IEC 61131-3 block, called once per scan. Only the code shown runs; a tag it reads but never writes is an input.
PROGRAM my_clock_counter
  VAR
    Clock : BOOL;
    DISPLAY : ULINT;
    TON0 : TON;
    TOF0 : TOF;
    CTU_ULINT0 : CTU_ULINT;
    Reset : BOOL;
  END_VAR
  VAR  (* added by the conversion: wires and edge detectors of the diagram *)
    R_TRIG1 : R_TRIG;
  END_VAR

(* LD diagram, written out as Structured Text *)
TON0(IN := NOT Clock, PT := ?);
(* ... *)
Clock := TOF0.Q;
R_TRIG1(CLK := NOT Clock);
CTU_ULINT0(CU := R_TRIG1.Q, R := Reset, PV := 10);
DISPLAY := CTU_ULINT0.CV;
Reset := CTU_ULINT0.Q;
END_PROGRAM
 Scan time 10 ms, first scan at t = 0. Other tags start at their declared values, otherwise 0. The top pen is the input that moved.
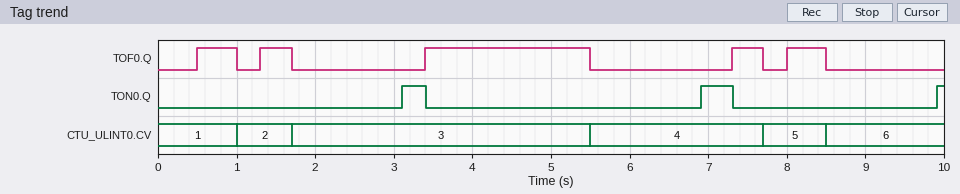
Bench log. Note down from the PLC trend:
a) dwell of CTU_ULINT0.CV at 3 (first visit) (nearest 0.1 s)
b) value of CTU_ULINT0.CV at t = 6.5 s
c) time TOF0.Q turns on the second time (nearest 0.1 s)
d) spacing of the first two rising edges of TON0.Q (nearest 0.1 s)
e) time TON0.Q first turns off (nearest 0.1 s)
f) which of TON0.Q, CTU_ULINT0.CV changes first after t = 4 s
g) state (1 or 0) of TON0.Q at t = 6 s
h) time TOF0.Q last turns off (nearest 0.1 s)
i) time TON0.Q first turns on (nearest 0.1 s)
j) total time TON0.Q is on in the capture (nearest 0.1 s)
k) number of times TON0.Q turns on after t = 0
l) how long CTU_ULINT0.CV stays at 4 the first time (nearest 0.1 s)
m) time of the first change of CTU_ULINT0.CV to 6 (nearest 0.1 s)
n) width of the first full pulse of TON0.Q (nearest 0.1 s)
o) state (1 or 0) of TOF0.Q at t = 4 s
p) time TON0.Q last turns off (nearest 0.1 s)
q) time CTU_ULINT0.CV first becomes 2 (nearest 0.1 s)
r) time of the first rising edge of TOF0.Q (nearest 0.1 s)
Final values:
3.8 s
4
1.3 s
3.8 s
3.4 s
CTU_ULINT0.CV
0
8.5 s
3.1 s
0.8 s
3
2.2 s
8.5 s
0.3 s
1
7.3 s
1.0 s
0.5 s
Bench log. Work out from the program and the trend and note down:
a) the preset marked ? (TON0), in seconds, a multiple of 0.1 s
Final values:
1.4 s
